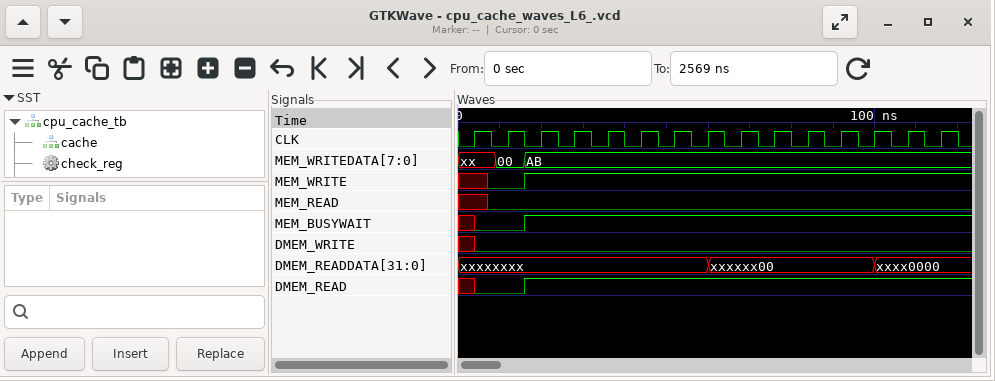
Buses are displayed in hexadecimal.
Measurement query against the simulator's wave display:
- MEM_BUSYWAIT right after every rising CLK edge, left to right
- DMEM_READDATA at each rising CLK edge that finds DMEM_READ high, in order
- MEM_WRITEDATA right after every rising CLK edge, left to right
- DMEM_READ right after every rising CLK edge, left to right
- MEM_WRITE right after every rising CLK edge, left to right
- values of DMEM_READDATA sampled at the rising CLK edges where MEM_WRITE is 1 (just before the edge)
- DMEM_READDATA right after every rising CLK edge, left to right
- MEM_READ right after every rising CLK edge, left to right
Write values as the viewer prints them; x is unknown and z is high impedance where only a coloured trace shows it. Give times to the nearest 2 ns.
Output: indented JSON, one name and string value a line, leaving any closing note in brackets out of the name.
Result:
{
  "MEM_BUSYWAIT right after every rising CLK edge, left to right": "0 0 1 1 1 1 1 1 1 1 1 1 1 1 1",
  "DMEM_READDATA at each rising CLK edge that finds DMEM_READ high, in order": "xxxxxxxx, xxxxxxxx, xxxxxxxx, xxxxxxxx, xxxxxxxx, xxxxxxxx, xxxxxx00, xxxxxx00, xxxxxx00, xxxxxx00, xxxxxx00, xxxx0000, xxxx0000",
  "MEM_WRITEDATA right after every rising CLK edge, left to right": "xx, 00, AB, AB, AB, AB, AB, AB, AB, AB, AB, AB, AB, AB, AB",
  "DMEM_READ right after every rising CLK edge, left to right": "0 0 1 1 1 1 1 1 1 1 1 1 1 1 1",
  "MEM_WRITE right after every rising CLK edge, left to right": "x 0 1 1 1 1 1 1 1 1 1 1 1 1 1",
  "values of DMEM_READDATA sampled at the rising CLK edges where MEM_WRITE is 1": "xxxxxxxx, xxxxxxxx, xxxxxxxx, xxxxxxxx, xxxxxxxx, xxxxxxxx, xxxxxx00, xxxxxx00, xxxxxx00, xxxxxx00, xxxxxx00, xxxx0000, xxxx0000",
  "DMEM_READDATA right after every rising CLK edge, left to right": "xxxxxxxx, xxxxxxxx, xxxxxxxx, xxxxxxxx, xxxxxxxx, xxxxxxxx, xxxxxxxx, xxxxxx00, xxxxxx00, xxxxxx00, xxxxxx00, xxxxxx00, xxxx0000, xxxx0000, xxxx0000",
  "MEM_READ right after every rising CLK edge, left to right": "x 0 0 0 0 0 0 0 0 0 0 0 0 0 0"
}
